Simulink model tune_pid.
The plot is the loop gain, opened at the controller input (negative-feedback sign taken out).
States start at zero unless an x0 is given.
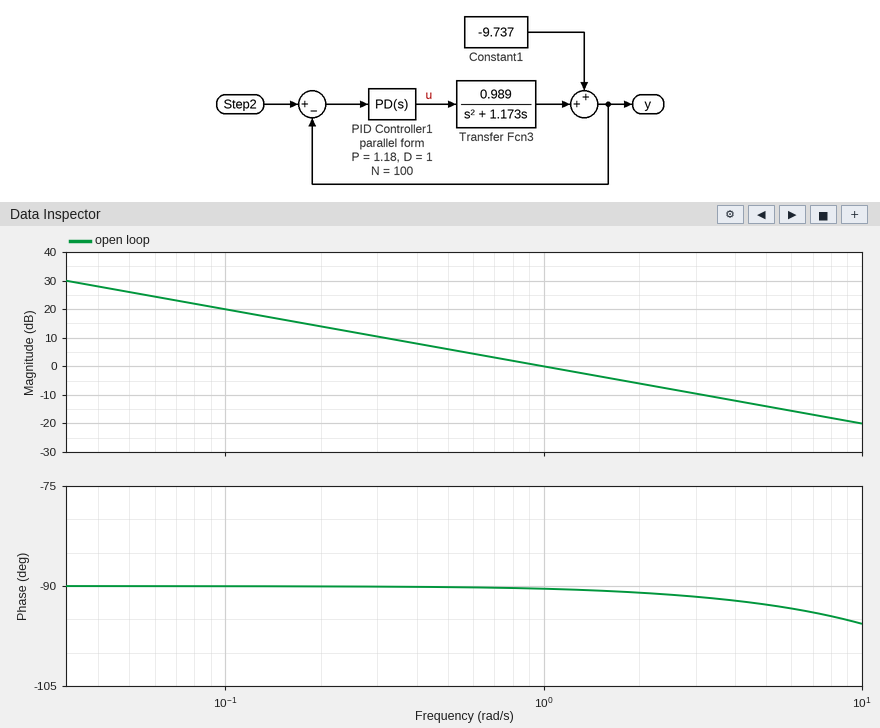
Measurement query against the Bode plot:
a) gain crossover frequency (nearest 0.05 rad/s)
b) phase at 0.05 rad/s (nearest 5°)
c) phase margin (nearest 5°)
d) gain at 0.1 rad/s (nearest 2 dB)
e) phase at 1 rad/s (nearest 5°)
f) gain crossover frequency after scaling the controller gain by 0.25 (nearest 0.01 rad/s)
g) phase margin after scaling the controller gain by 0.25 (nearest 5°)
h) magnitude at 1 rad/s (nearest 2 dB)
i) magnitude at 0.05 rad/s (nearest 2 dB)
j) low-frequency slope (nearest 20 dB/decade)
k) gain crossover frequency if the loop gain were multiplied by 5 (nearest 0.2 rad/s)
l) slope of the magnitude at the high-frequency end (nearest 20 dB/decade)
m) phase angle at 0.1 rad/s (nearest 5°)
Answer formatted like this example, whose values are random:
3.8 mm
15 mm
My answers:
1.00 rad/s
-90°
90°
20 dB
-90°
0.25 rad/s
90°
0 dB
26 dB
-20 dB/decade
5.0 rad/s
-20 dB/decade
-90°
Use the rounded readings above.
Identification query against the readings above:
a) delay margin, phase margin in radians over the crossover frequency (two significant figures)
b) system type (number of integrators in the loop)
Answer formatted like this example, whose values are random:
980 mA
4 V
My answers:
1.6 s
1
